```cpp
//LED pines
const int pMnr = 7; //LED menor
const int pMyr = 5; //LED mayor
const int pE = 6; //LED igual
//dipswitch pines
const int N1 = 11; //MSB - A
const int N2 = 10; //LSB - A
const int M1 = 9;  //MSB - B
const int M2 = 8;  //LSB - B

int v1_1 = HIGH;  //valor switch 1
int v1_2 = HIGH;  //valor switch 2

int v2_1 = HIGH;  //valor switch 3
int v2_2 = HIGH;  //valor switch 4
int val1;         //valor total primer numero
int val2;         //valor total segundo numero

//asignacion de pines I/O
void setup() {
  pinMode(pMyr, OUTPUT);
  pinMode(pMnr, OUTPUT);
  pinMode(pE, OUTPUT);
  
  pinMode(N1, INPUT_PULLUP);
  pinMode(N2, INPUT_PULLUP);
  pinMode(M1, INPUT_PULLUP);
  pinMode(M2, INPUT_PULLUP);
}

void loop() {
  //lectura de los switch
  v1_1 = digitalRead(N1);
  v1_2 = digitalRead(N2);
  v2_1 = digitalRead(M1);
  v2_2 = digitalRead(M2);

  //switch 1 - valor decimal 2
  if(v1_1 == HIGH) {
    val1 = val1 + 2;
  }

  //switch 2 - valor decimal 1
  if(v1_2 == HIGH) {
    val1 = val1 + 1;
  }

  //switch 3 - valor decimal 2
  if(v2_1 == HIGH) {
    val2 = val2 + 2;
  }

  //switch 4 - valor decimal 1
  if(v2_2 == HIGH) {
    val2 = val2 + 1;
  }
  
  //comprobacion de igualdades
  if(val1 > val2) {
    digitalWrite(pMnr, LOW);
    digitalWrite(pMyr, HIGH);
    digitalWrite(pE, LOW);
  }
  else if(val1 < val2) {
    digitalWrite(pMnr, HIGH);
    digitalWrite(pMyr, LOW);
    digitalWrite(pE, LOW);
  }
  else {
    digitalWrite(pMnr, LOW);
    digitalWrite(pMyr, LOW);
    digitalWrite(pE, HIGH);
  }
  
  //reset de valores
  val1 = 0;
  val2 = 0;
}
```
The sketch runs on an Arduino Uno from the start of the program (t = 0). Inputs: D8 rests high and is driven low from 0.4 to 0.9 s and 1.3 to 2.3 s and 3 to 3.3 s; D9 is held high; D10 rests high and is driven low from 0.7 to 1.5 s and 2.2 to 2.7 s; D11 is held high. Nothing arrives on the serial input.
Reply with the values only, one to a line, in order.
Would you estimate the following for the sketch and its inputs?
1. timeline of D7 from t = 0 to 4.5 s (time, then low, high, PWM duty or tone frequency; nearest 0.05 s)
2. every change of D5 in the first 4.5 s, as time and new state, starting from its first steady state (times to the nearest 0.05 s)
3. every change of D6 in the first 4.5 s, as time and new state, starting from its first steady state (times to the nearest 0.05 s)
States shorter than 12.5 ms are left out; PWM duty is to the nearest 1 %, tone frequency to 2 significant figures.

0 s low; 0.9 s high; 1.3 s low; 2.3 s high; 2.7 s low
0 s low; 0.4 s high; 0.7 s low; 1.5 s high; 2.2 s low; 3 s high; 3.3 s low
0 s high; 0.4 s low; 0.7 s high; 0.9 s low; 1.3 s high; 1.5 s low; 2.2 s high; 2.3 s low; 2.7 s high; 3 s low; 3.3 s high
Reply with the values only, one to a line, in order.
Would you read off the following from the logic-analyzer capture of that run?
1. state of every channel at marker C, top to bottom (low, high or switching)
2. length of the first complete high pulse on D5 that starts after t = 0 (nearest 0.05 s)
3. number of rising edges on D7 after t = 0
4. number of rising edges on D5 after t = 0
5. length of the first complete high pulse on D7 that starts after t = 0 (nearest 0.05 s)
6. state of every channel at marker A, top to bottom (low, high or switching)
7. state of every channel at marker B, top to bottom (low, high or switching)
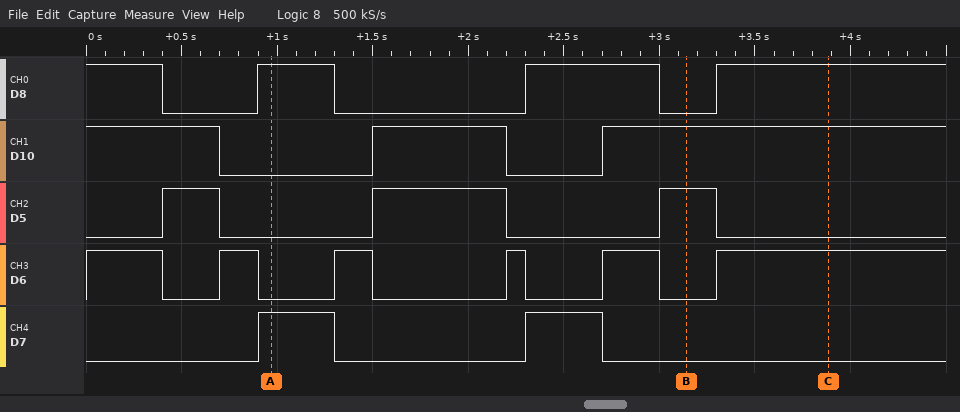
D8 high, D10 high, D5 low, D6 high, D7 low
0.30 s
2
3
0.40 s
D8 high, D10 low, D5 low, D6 low, D7 high
D8 low, D10 high, D5 high, D6 low, D7 low
